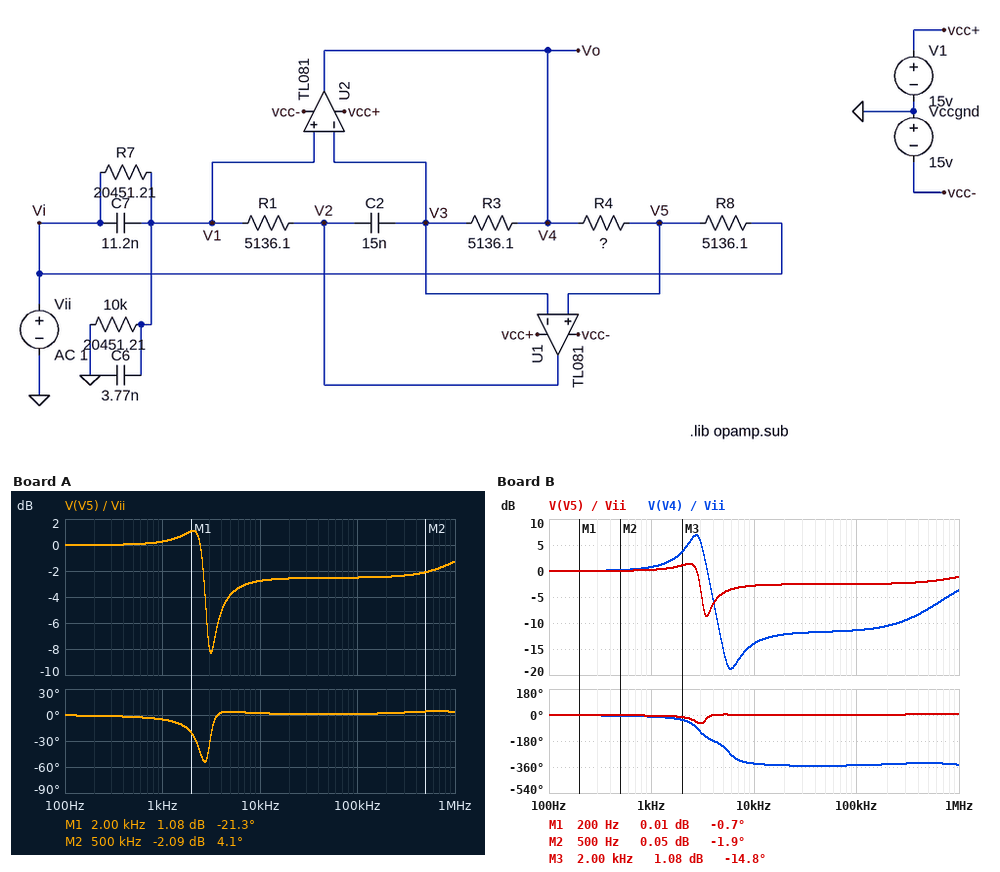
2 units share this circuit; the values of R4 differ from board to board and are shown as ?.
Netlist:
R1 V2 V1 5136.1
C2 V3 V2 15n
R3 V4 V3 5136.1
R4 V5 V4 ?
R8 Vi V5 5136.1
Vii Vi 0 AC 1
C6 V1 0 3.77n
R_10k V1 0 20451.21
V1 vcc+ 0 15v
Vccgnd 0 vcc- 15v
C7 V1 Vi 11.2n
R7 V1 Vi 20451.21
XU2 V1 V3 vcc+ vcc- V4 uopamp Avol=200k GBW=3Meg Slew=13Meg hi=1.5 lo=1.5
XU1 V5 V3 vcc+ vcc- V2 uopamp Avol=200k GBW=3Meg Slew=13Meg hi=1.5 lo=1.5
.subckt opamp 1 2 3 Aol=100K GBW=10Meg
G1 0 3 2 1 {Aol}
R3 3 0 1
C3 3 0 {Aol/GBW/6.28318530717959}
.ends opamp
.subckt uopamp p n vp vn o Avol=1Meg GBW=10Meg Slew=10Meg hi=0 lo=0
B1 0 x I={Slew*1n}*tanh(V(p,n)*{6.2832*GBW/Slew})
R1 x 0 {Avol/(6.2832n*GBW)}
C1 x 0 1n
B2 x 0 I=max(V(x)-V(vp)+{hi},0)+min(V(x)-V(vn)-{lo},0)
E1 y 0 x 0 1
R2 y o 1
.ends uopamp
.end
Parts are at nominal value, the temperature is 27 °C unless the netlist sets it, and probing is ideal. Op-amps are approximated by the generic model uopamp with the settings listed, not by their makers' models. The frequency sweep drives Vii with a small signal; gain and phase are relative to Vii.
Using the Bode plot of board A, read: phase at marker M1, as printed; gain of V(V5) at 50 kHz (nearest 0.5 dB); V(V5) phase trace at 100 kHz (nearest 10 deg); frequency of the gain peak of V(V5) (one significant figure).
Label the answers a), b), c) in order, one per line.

a) -21.3 deg
b) -2.5 dB
c) 0 deg
d) 2 kHz
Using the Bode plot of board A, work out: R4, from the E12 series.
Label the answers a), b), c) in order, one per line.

a) 8.2 kΩ
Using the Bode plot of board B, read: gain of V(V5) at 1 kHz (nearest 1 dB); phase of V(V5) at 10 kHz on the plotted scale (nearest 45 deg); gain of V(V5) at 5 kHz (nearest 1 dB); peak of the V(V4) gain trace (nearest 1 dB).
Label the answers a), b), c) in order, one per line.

a) 0 dB
b) 0 deg
c) -4 dB
d) 7 dB
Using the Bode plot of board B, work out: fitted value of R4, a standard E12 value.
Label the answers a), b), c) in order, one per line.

a) 10 kΩ
